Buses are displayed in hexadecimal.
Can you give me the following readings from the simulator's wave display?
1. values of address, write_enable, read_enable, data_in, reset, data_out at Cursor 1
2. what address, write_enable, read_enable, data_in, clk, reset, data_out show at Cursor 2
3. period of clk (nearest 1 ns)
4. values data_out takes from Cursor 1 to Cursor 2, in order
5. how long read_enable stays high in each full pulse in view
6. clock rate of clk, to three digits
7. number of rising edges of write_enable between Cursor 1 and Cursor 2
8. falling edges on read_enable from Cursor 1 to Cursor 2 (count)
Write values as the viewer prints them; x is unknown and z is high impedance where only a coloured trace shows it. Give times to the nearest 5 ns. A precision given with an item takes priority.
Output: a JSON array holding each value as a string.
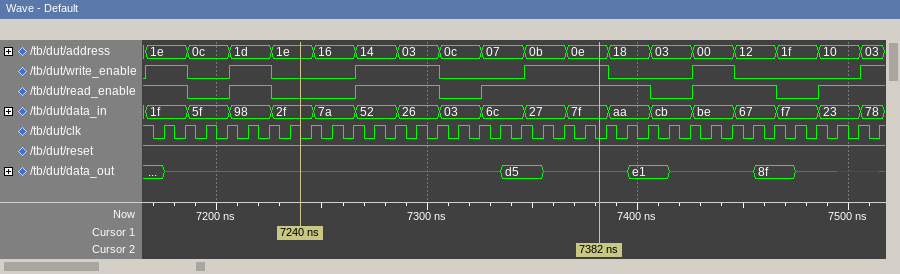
["address=1e, write_enable=0, read_enable=0, data_in=2f, reset=1, data_out=z", "address=0e, write_enable=1, read_enable=1, data_in=7f, clk=0, reset=1, data_out=z", "10 ns", "z, d5, z", "20 ns, 40 ns, 80 ns, 40 ns", "100 MHz", "2", "1"]
